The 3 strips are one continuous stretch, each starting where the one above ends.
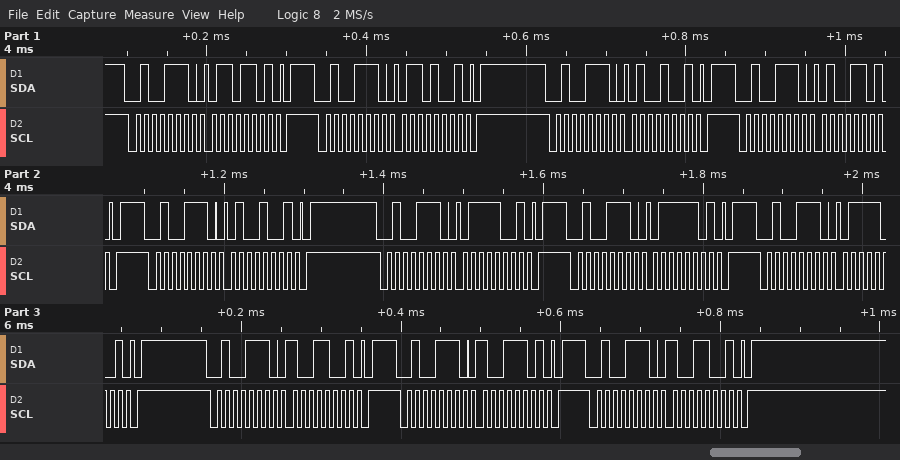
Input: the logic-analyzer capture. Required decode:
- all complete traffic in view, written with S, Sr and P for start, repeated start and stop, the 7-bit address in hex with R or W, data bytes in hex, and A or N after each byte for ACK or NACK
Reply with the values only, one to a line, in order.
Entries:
S 27W A 6D A P S 27W A 69 A P S 27W A 49 A P S 27W A 4D A P S 27W A 49 A P S 27W A 79 A P S 27W A 7D A P S 27W A 79 A P S 27W A 99 A P S 27W A 9D A P S 27W A 99 A P
